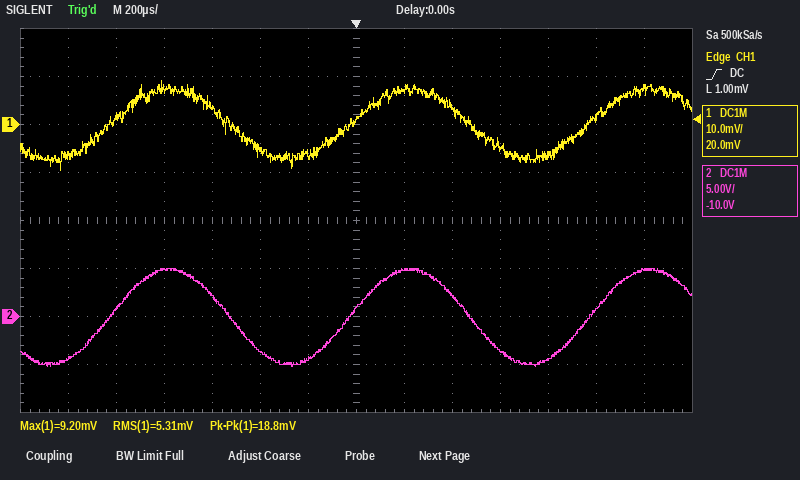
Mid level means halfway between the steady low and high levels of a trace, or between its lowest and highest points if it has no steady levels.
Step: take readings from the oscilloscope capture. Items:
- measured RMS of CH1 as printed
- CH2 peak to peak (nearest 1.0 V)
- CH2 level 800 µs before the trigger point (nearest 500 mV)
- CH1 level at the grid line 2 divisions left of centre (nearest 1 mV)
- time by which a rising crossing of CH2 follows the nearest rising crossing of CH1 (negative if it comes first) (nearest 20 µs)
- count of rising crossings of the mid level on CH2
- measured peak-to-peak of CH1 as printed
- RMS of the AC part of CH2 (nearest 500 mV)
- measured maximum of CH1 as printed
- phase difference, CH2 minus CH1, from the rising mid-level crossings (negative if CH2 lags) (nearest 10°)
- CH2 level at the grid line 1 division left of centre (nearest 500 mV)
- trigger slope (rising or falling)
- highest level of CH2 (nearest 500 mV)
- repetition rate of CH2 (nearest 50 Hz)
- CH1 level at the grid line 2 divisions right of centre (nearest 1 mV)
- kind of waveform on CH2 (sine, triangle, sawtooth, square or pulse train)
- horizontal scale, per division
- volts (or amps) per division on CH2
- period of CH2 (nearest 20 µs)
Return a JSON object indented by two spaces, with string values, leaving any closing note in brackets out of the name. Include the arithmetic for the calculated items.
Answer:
{
  "measured RMS of CH1 as printed": "5.31 mV",
  "CH2 peak to peak": "10.0 V",
  "CH2 level 800 µs before the trigger point": "5.0 V",
  "CH1 level at the grid line 2 divisions left of centre": "-5 mV",
  "time by which a rising crossing of CH2 follows the nearest rising crossing of CH1 (negative if it comes first)": "0 µs",
  "count of rising crossings of the mid level on CH2": "3",
  "measured peak-to-peak of CH1 as printed": "18.8 mV",
  "RMS of the AC part of CH2": "10.0 V / (2√2) ≈ 3.5 V",
  "measured maximum of CH1 as printed": "9.20 mV",
  "phase difference, CH2 minus CH1, from the rising mid-level crossings (negative if CH2 lags)": "−360° × (0 µs) / 1.00 ms ≈ 0°",
  "CH2 level at the grid line 1 division left of centre": "-4.5 V",
  "trigger slope": "rising",
  "highest level of CH2": "5.0 V",
  "repetition rate of CH2": "1 / 1.00 ms ≈ 1.00 kHz",
  "CH1 level at the grid line 2 divisions right of centre": "4 mV",
  "kind of waveform on CH2": "sine",
  "horizontal scale, per division": "200 µs",
  "volts (or amps) per division on CH2": "5 V",
  "period of CH2": "1.00 ms"
}
